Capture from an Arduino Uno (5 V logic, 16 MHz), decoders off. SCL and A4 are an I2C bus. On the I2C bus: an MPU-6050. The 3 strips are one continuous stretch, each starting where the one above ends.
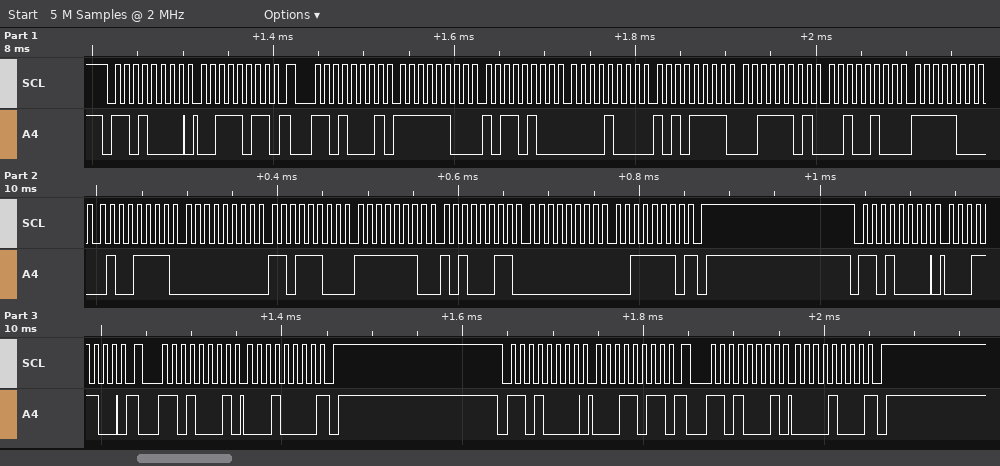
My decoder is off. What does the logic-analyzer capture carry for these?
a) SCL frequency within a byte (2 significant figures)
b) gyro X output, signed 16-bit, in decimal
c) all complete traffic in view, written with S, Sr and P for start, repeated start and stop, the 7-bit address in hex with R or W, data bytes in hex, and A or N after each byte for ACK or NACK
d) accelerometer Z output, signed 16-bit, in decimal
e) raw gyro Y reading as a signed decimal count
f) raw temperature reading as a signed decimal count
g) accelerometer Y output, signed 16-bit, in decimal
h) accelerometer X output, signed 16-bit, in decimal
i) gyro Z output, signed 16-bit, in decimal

100 kHz
220
S 68W A 3B A Sr 68R A FC A B4 A 08 A AF A 3D A 24 A F8 A 4F A 00 A DC A FE A A3 A 00 A 3E N P S 68W A 1C A Sr 68R A 10 N P S 68W A 1B A Sr 68R A 08 N P
15652
-349
-1969
2223
-844
62
